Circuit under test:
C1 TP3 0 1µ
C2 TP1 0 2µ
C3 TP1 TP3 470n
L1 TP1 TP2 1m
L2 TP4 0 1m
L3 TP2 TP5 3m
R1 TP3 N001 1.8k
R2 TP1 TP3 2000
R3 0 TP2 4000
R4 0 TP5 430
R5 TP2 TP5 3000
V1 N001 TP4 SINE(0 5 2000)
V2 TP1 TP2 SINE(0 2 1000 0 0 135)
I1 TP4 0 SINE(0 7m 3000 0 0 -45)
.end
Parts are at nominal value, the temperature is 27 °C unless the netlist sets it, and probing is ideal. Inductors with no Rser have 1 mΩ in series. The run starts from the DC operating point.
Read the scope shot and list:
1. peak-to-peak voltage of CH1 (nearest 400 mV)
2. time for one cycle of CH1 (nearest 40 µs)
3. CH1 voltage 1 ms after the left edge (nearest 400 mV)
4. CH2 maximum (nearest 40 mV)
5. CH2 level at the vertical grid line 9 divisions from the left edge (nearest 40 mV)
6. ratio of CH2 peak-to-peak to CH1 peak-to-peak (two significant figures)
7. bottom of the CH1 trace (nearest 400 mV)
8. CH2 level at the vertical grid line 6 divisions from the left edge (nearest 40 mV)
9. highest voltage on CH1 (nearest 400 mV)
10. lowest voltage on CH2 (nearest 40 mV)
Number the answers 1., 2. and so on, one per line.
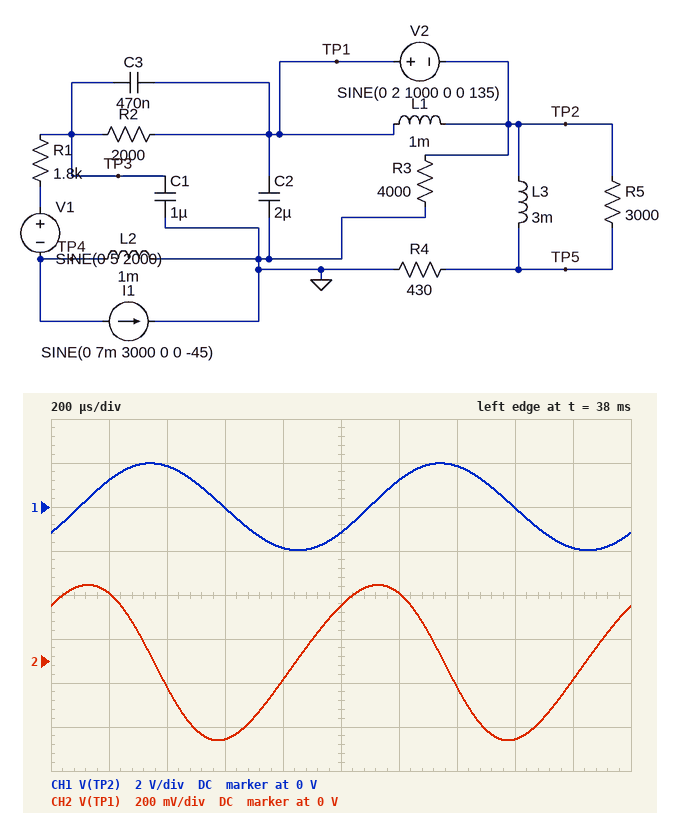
1. 4.0 V
2. 1.00 ms
3. -1.2 V
4. 360 mV
5. -80 mV
6. 0.18
7. -2.0 V
8. 320 mV
9. 2.0 V
10. -360 mV
